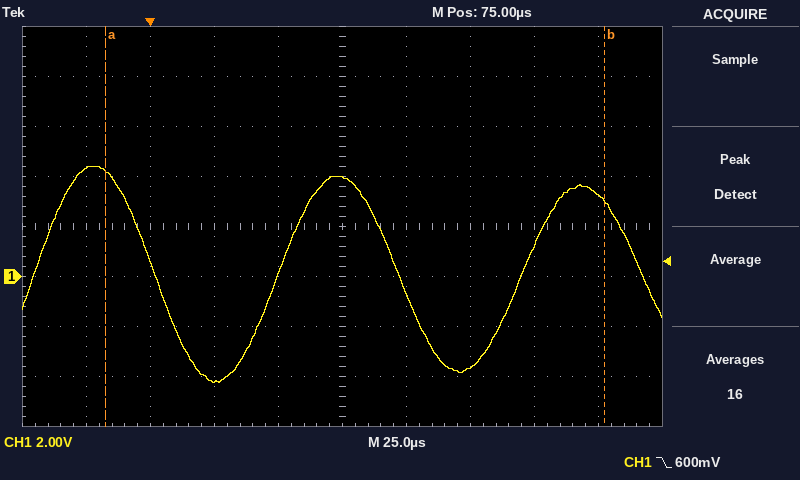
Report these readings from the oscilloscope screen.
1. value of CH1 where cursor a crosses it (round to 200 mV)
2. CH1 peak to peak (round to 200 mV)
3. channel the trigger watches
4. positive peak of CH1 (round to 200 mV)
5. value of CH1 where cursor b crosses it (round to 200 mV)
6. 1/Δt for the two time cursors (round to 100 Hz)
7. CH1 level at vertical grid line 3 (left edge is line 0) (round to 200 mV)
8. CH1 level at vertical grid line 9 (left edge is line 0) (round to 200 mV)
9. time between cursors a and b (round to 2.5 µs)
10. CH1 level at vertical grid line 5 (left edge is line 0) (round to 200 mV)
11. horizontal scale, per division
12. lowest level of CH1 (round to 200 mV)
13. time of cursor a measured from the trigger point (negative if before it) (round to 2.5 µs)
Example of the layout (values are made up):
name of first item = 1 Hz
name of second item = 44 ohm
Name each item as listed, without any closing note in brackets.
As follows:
value of CH1 where cursor a crosses it = 4.2 V
CH1 peak to peak = 8.6 V
channel the trigger watches = CH1
positive peak of CH1 = 4.4 V
value of CH1 where cursor b crosses it = 3.0 V
1/Δt for the two time cursors = 5.1 kHz
CH1 level at vertical grid line 3 (left edge is line 0) = -4.2 V
CH1 level at vertical grid line 9 (left edge is line 0) = 3.2 V
time between cursors a and b = 195.0 µs
CH1 level at vertical grid line 5 (left edge is line 0) = 4.0 V
horizontal scale, per division = 25 µs
lowest level of CH1 = -4.2 V
time of cursor a measured from the trigger point (negative if before it) = -17.5 µs
